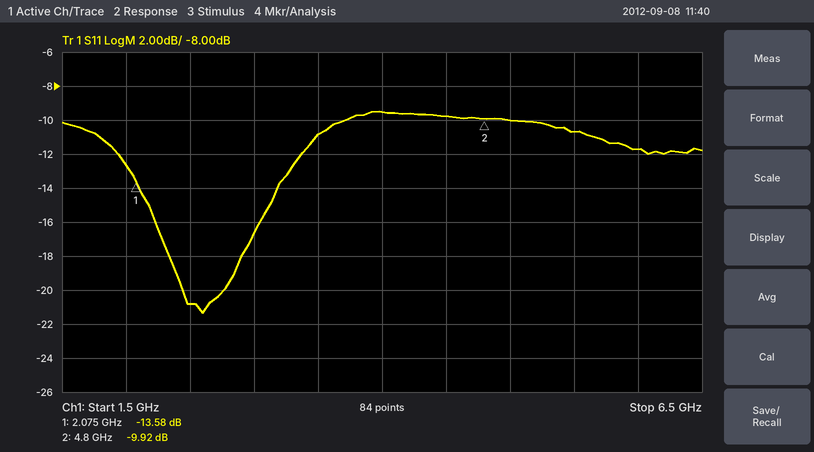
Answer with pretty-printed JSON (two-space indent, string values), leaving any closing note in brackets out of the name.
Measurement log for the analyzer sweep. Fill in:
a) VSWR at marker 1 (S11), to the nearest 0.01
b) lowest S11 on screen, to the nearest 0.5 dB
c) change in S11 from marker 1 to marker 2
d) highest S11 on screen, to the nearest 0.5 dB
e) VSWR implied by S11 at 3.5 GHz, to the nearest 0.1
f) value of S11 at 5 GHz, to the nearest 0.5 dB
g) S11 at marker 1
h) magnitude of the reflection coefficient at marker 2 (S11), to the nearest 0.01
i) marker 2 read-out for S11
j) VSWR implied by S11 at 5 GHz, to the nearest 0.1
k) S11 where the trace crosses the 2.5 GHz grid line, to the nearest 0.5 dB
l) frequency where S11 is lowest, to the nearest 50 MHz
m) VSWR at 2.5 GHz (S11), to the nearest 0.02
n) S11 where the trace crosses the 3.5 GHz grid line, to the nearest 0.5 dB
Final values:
{
  "VSWR at marker 1 (S11), to the nearest 0.01": "1.53",
  "lowest S11 on screen, to the nearest 0.5 dB": "-21.5 dB",
  "change in S11 from marker 1 to marker 2": "3.66 dB",
  "highest S11 on screen, to the nearest 0.5 dB": "-9.5 dB",
  "VSWR implied by S11 at 3.5 GHz, to the nearest 0.1": "1.8",
  "value of S11 at 5 GHz, to the nearest 0.5 dB": "-10.0 dB",
  "S11 at marker 1": "-13.58 dB",
  "magnitude of the reflection coefficient at marker 2 (S11), to the nearest 0.01": "0.32",
  "marker 2 read-out for S11": "-9.92 dB",
  "VSWR implied by S11 at 5 GHz, to the nearest 0.1": "1.9",
  "S11 where the trace crosses the 2.5 GHz grid line, to the nearest 0.5 dB": "-21.0 dB",
  "frequency where S11 is lowest, to the nearest 50 MHz": "2.60 GHz",
  "VSWR at 2.5 GHz (S11), to the nearest 0.02": "1.20",
  "S11 where the trace crosses the 3.5 GHz grid line, to the nearest 0.5 dB": "-11.0 dB"
}
